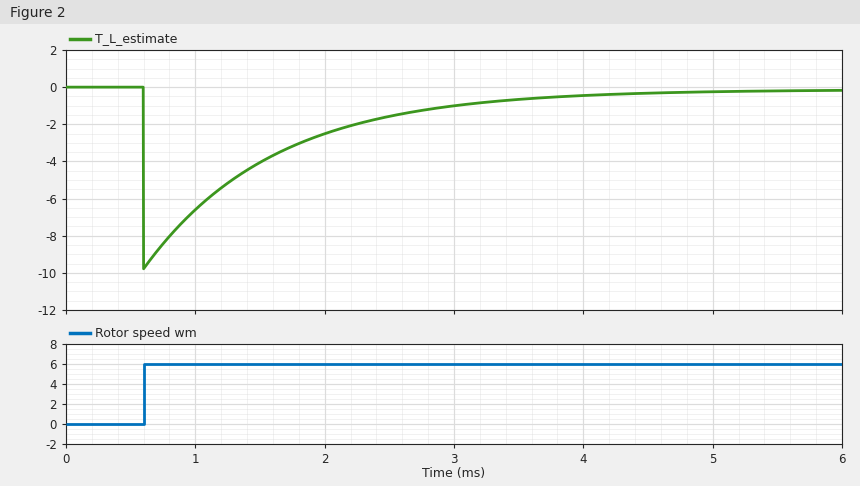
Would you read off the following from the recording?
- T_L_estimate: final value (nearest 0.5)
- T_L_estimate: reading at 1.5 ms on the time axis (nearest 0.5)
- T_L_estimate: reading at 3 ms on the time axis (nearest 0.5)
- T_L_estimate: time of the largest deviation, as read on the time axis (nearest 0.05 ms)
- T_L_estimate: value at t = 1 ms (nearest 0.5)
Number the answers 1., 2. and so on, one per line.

1. 0.0
2. -4.0
3. -1.0
4. 0.60 ms
5. -6.5
